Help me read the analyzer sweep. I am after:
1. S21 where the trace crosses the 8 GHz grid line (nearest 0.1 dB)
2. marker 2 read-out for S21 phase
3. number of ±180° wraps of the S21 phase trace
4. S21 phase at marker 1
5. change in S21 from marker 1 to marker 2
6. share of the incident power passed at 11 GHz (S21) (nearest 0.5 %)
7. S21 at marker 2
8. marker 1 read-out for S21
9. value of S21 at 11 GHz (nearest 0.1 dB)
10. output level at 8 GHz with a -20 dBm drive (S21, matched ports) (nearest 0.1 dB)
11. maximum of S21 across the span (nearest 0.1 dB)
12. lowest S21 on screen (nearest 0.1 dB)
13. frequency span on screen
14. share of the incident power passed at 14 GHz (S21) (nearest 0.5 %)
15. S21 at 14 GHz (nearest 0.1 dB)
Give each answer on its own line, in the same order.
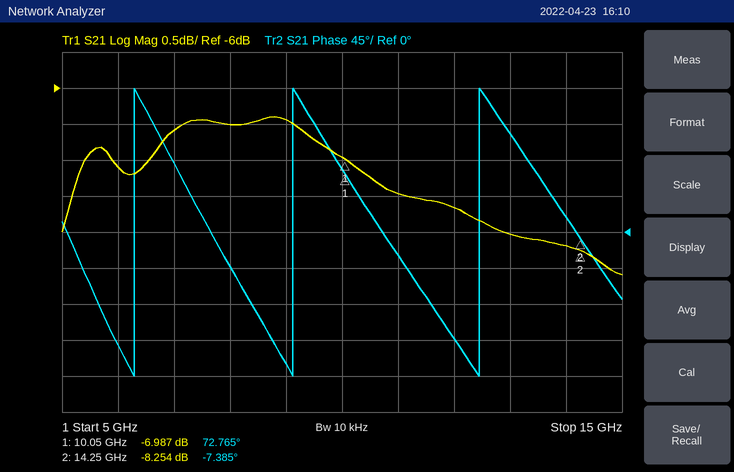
-6.5 dB
-7.385°
3
72.765°
-1.267 dB
18.0 %
-8.254 dB
-6.987 dB
-7.5 dB
-26.5 dBm
-6.4 dB
-8.6 dB
10 GHz
15.0 %
-8.2 dB
